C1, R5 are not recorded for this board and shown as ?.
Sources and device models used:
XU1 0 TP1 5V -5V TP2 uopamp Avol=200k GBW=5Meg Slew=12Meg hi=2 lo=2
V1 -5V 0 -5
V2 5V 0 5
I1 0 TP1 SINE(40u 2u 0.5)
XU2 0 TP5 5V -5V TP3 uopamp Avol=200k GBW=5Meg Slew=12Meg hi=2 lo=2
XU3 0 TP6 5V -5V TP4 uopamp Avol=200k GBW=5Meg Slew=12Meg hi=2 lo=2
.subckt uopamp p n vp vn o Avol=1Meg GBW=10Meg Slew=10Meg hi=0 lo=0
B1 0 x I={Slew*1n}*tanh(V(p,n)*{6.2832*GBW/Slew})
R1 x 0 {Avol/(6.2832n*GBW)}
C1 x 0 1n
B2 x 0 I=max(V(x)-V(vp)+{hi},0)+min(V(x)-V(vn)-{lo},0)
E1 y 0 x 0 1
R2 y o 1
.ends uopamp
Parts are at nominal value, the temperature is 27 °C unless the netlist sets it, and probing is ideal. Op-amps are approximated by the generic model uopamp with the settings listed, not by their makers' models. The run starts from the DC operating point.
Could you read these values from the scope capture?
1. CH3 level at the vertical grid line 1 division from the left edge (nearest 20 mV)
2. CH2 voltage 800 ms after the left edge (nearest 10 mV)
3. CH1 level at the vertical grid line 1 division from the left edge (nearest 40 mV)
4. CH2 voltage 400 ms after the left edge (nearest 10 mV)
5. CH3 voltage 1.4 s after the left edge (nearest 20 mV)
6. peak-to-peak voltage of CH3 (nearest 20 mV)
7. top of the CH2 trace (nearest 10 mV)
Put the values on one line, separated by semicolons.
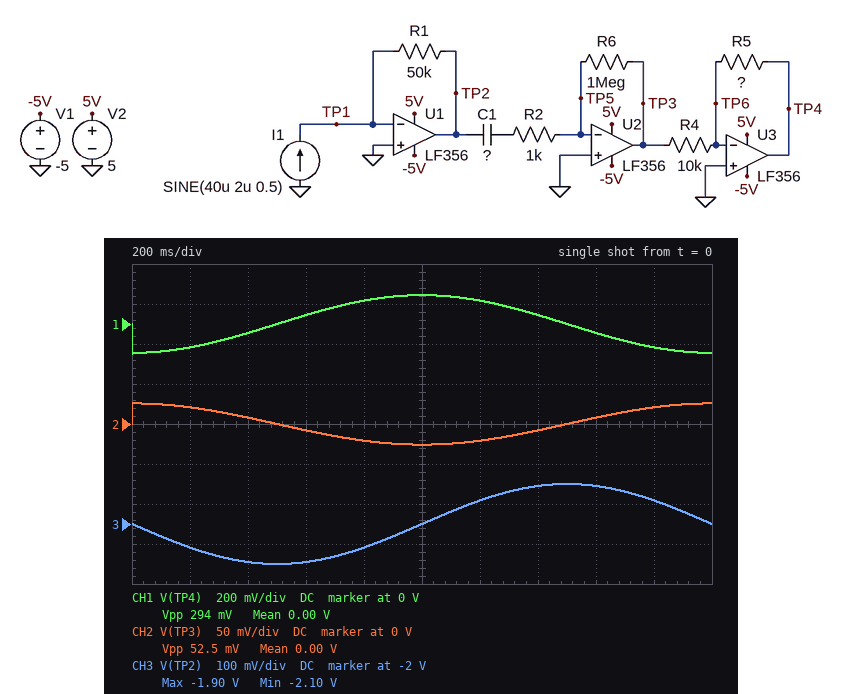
-2.06 V; -20 mV; -120 mV; 10 mV; -1.90 V; 200 mV; 30 mV
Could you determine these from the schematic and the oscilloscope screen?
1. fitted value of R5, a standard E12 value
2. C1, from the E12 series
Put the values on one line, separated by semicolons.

56 kΩ; 82 nF
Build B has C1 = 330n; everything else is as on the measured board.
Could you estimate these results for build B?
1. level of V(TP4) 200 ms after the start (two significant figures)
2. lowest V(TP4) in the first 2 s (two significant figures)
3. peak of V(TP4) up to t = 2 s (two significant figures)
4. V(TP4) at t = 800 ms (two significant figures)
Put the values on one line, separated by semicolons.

-470 mV; -580 mV; 580 mV; 470 mV
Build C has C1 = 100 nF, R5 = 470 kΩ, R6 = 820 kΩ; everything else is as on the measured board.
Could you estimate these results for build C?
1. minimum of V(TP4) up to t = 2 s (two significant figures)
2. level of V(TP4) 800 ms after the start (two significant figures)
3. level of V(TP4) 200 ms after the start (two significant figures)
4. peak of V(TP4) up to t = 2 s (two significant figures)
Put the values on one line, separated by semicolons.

-1.2 V; 980 mV; -980 mV; 1.2 V
